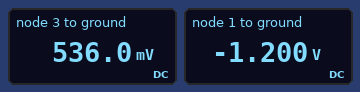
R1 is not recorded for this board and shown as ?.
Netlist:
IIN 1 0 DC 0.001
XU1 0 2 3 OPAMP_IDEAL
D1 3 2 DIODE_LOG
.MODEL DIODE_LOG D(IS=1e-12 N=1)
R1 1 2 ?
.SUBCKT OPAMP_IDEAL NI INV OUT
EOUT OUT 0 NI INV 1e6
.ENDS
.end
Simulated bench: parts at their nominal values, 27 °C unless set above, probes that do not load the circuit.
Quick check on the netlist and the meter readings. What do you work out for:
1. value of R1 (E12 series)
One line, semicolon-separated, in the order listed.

1.2 kΩ
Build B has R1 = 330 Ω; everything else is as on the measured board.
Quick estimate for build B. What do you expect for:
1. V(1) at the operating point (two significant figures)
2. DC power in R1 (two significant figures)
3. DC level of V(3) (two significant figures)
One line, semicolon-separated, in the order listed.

-330 mV; 330 µW; 540 mV
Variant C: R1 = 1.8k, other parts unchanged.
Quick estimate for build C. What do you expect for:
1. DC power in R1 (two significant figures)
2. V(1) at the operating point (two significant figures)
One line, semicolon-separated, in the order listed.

1.8 mW; -1.8 V
